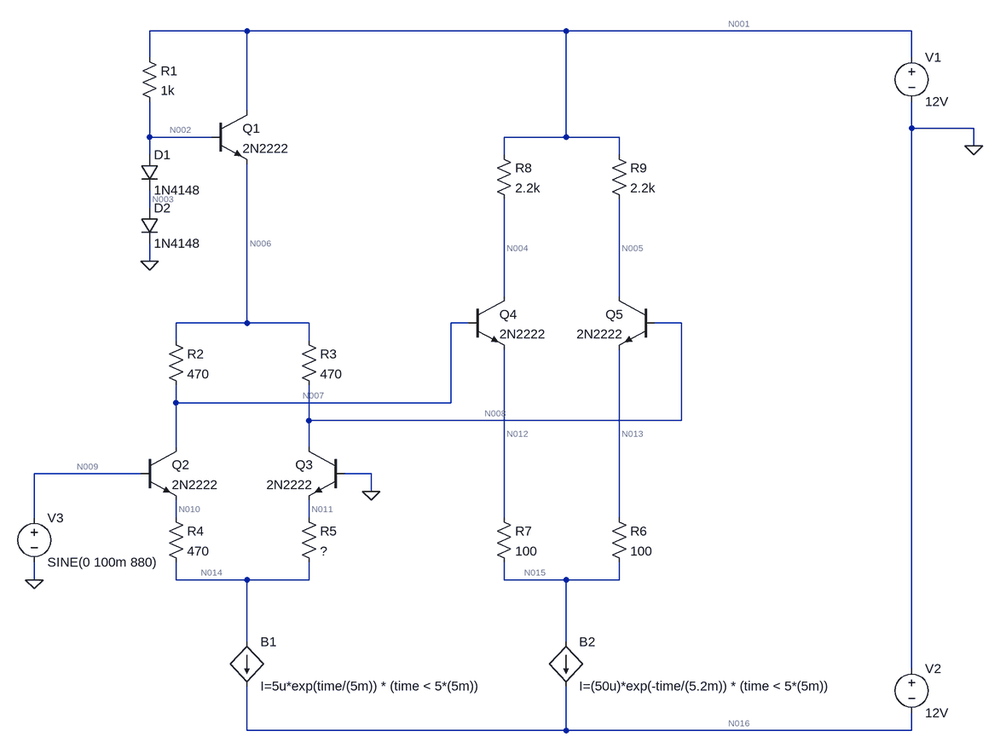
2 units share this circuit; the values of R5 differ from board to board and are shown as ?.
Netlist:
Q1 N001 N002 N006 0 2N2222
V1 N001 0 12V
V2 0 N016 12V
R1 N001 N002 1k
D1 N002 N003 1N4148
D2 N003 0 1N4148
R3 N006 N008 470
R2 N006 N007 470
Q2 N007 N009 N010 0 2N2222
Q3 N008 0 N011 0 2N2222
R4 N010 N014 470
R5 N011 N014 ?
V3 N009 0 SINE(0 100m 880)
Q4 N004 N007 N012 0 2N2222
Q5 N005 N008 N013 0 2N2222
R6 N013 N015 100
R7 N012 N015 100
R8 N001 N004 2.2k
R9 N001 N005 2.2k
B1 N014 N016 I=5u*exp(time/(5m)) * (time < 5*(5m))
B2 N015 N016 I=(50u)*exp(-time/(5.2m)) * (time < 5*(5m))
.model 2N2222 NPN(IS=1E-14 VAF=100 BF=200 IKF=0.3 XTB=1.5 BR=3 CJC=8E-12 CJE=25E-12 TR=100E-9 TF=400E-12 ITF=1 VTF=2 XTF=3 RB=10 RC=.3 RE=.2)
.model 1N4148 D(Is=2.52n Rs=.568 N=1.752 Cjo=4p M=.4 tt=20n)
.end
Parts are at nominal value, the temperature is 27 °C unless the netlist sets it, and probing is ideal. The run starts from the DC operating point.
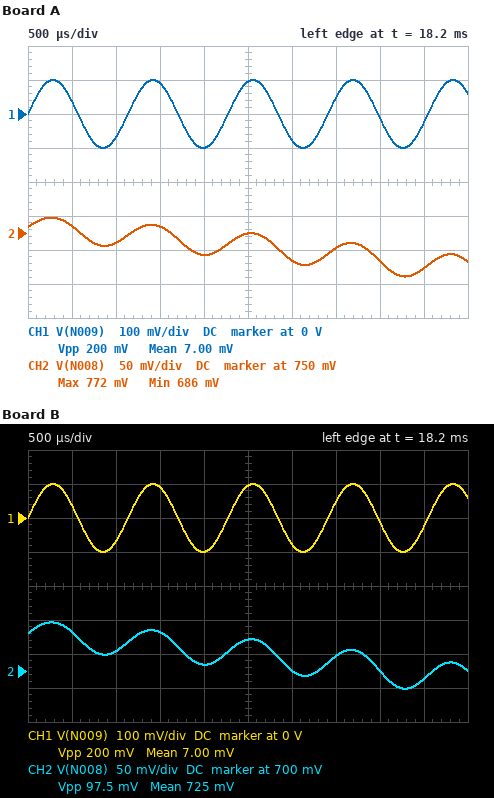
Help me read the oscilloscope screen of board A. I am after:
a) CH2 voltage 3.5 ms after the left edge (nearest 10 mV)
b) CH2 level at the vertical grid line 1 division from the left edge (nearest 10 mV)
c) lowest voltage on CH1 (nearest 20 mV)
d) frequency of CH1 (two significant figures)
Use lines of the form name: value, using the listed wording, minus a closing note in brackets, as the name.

CH2 voltage 3.5 ms after the left edge: 730 mV
CH2 level at the vertical grid line 1 division from the left edge: 760 mV
lowest voltage on CH1: -100 mV
frequency of CH1: 880 Hz
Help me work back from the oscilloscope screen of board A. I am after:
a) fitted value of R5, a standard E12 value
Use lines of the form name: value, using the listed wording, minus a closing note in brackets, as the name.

fitted value of R5, a standard E12 value: 1.5 kΩ
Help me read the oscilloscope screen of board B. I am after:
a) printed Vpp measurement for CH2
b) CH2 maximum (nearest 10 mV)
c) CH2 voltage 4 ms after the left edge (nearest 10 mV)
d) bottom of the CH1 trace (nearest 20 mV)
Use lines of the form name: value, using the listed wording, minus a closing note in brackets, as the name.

printed Vpp measurement for CH2: 97.5 mV
CH2 maximum: 770 mV
CH2 voltage 4 ms after the left edge: 700 mV
bottom of the CH1 trace: -100 mV
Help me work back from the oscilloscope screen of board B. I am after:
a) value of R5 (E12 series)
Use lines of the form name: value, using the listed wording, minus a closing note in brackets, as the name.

value of R5: 1.2 kΩ
